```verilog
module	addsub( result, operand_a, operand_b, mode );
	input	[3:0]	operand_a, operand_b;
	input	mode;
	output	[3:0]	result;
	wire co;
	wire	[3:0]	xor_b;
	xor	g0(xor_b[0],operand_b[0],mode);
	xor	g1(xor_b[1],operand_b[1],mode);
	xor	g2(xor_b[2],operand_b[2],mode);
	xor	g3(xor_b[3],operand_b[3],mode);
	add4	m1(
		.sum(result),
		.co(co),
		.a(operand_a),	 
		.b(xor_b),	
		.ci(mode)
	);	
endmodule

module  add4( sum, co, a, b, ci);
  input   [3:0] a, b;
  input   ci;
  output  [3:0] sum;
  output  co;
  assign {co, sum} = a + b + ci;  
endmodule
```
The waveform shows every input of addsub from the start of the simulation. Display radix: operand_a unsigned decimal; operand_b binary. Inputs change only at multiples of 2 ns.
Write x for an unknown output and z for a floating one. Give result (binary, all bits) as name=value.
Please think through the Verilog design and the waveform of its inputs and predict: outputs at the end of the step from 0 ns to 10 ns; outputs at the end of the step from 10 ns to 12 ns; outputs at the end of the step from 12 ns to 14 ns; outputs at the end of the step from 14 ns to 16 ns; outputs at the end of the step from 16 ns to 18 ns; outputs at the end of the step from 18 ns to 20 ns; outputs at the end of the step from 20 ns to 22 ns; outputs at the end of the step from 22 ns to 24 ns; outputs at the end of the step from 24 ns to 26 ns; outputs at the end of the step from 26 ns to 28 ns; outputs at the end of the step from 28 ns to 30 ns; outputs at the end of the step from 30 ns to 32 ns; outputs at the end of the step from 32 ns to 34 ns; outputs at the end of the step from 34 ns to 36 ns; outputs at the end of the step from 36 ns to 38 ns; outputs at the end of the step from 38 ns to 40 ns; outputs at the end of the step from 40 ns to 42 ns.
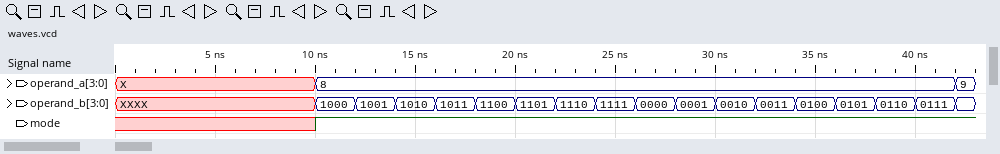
result=x
result=0000
result=1111
result=1110
result=1101
result=1100
result=1011
result=1010
result=1001
result=1000
result=0111
result=0110
result=0101
result=0100
result=0011
result=0010
result=0001
